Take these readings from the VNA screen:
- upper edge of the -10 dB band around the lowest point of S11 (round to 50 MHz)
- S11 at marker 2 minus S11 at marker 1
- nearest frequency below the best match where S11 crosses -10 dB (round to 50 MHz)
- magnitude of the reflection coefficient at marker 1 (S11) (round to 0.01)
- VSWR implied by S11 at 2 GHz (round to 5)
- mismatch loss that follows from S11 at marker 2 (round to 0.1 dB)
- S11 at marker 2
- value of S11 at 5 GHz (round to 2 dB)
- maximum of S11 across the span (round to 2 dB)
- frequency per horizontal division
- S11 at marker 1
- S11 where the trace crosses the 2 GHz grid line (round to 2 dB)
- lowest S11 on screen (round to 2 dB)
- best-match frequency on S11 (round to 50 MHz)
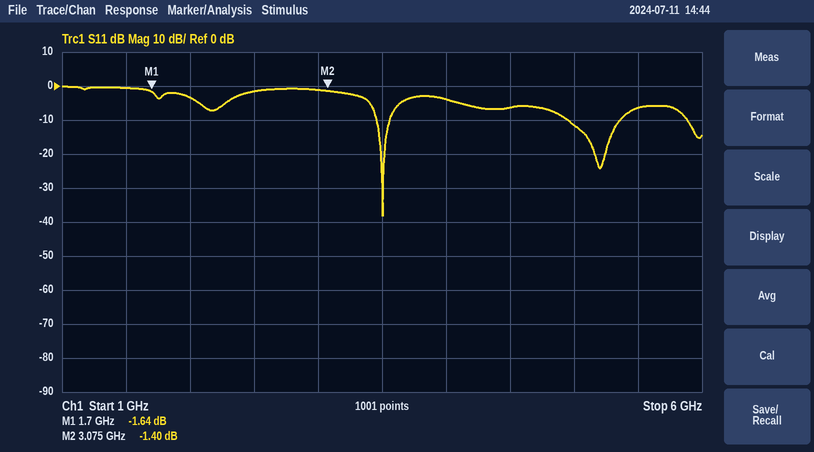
3.55 GHz
0.24 dB
3.45 GHz
0.83
5
5.6 dB
-1.40 dB
-12 dB
0 dB
500 MHz
-1.64 dB
-4 dB
-38 dB
3.50 GHz
